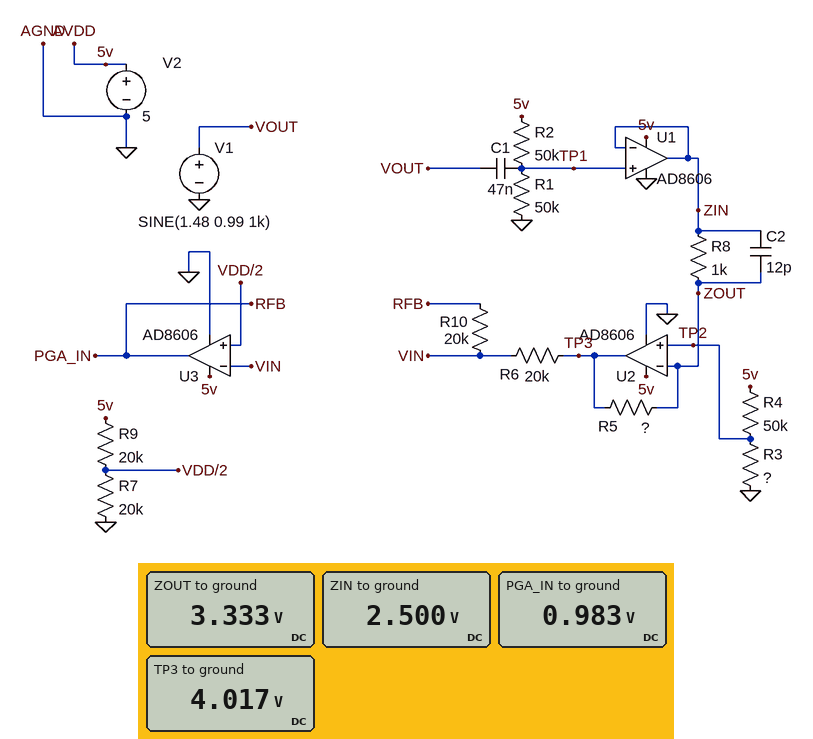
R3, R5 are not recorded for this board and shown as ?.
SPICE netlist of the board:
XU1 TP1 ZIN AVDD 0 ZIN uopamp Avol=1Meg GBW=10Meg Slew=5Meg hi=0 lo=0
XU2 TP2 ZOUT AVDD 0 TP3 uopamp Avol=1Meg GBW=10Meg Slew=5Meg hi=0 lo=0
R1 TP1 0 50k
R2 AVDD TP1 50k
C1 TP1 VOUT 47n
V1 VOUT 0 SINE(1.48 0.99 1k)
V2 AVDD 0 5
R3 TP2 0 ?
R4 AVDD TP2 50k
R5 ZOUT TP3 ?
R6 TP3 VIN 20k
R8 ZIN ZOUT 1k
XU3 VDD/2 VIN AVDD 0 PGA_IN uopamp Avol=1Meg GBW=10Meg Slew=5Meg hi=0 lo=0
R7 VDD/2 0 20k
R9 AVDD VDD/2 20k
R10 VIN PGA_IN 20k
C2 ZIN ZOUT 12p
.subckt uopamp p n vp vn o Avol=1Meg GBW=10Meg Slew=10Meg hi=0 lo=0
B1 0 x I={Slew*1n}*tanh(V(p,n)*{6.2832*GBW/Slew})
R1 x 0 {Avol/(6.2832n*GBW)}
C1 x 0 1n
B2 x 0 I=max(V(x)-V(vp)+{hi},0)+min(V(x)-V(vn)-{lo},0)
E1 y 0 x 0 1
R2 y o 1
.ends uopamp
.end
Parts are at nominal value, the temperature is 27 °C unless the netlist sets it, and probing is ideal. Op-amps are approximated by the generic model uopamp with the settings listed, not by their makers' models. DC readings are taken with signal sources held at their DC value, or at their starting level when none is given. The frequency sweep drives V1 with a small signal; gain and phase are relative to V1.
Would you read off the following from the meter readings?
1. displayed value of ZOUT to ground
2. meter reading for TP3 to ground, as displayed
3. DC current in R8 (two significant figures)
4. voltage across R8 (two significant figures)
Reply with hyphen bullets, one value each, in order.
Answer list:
- 3.333 V
- 4.017 V
- 830 µA
- 830 mV
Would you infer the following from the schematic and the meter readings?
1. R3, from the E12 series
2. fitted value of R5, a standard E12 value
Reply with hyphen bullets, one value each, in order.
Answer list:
- 100 kΩ
- 820 Ω
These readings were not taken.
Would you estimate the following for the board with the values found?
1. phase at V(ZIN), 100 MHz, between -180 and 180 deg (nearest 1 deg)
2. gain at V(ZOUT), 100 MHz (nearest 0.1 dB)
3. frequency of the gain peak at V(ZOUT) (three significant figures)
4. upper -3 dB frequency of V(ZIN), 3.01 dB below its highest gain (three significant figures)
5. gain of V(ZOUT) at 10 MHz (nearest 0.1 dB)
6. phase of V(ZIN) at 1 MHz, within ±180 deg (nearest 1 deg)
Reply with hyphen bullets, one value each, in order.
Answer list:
- -84 deg
- -20.2 dB
- 10.5 MHz
- 9.99 MHz
- -8.2 dB
- -6 deg
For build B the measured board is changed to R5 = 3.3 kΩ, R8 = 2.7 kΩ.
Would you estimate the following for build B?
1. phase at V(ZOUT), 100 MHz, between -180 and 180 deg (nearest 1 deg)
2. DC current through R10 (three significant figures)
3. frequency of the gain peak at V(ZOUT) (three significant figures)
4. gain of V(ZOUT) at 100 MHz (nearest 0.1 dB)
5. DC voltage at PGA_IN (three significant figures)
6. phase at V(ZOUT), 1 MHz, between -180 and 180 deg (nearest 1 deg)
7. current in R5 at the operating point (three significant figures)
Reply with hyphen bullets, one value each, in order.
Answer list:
- -82 deg
- 92.6 µA
- 7.55 MHz
- -20.0 dB
- 648 mV
- 83 deg
- 309 µA
